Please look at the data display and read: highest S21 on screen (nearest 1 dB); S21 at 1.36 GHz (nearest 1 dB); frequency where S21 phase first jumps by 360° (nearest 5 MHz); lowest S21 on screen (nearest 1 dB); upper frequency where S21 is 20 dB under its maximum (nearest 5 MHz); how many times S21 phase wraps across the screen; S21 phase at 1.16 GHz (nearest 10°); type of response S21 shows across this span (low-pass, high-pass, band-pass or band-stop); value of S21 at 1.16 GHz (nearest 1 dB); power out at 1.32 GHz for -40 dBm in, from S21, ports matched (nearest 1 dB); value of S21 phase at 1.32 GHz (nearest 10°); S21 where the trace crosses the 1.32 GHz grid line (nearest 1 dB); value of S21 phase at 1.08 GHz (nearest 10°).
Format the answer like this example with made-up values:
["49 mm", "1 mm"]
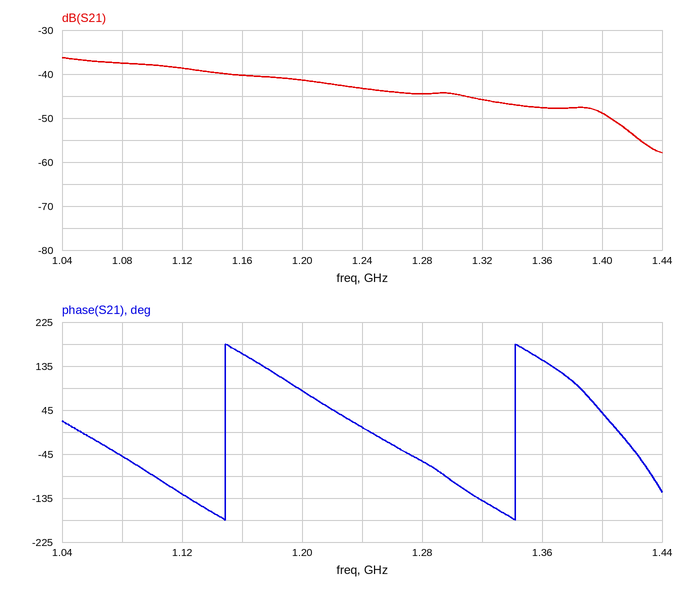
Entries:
["-36 dB", "-48 dB", "1.150 GHz", "-58 dB", "1.430 GHz", "2", "160°", "low-pass", "-40 dB", "-86 dBm", "-140°", "-46 dB", "-50°"]
